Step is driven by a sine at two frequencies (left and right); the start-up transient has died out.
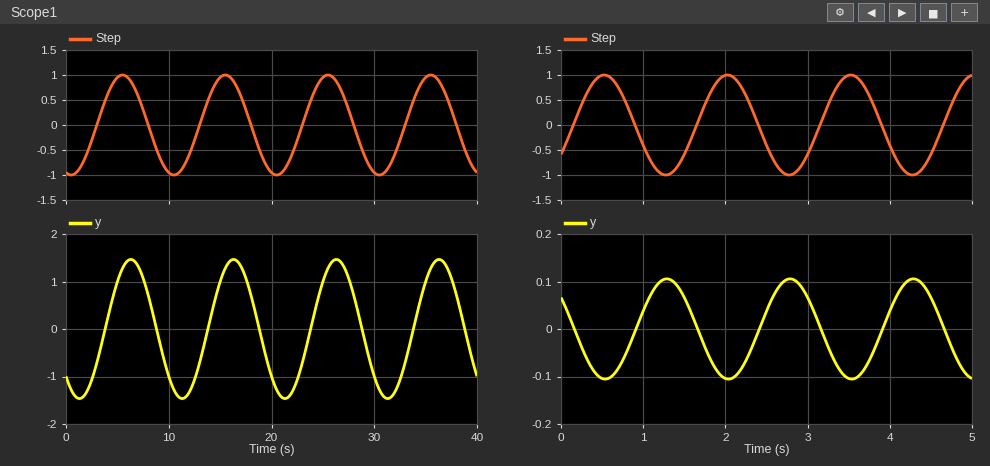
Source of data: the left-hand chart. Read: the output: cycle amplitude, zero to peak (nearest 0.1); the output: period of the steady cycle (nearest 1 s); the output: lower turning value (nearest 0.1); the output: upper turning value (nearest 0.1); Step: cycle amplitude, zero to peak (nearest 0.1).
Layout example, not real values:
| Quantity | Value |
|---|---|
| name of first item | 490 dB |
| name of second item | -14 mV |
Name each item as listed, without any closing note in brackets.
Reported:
| Quantity | Value |
|---|---|
| the output: cycle amplitude, zero to peak | 1.5 |
| the output: period of the steady cycle | 10 s |
| the output: lower turning value | -1.5 |
| the output: upper turning value | 1.5 |
| Step: cycle amplitude, zero to peak | 1.0 |
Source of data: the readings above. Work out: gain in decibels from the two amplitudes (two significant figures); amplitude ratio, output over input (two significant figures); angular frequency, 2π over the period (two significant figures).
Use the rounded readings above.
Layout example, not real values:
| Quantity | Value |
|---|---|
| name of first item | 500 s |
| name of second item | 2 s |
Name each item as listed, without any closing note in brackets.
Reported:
| Quantity | Value |
|---|---|
| gain in decibels from the two amplitudes | 3.5 dB |
| amplitude ratio, output over input | 1.5 |
| angular frequency, 2π over the period | 0.63 rad/s |
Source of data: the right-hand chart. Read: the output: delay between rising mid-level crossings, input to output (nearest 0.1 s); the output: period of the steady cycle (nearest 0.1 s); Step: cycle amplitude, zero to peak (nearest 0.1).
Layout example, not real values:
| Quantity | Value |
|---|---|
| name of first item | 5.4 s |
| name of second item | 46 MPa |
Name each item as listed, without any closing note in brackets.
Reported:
| Quantity | Value |
|---|---|
| the output: delay between rising mid-level crossings, input to output | 0.8 s |
| the output: period of the steady cycle | 1.5 s |
| Step: cycle amplitude, zero to peak | 1.0 |
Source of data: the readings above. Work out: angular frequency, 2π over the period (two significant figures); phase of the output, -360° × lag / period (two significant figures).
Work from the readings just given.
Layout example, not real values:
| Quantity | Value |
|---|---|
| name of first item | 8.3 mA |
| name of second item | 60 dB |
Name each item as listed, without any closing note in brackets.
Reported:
| Quantity | Value |
|---|---|
| angular frequency, 2π over the period | 4.2 rad/s |
| phase of the output, -360° × lag / period | -190° |
